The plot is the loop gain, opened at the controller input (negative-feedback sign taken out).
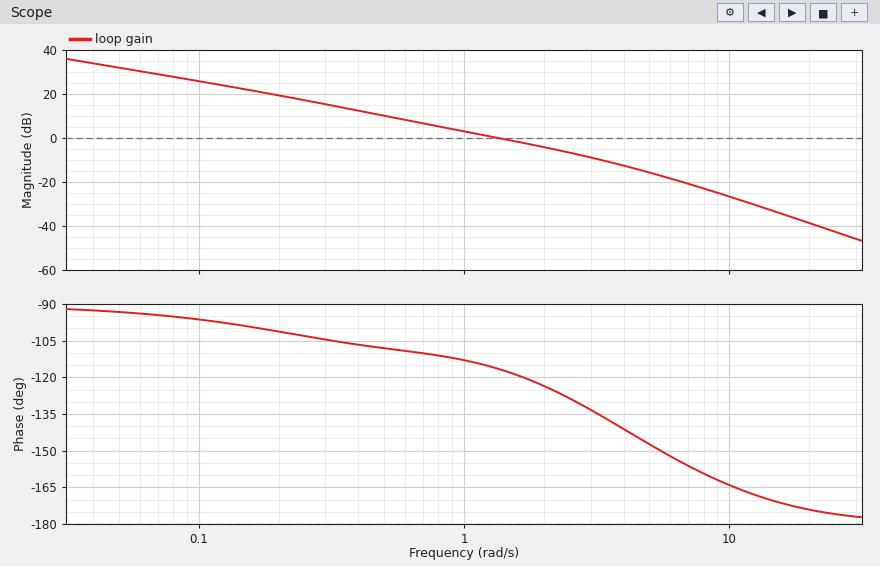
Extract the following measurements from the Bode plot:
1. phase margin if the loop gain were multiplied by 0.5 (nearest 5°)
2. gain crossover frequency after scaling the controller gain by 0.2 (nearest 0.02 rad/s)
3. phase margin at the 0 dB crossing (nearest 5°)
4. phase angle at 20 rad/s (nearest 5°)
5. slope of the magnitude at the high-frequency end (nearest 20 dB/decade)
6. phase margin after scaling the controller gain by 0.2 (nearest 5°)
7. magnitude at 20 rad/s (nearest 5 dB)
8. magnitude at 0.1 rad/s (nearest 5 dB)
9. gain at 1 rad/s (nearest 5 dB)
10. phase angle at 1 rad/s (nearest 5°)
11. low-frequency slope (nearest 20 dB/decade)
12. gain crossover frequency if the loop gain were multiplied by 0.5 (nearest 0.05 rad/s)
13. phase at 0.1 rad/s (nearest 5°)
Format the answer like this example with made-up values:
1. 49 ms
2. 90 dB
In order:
1. 70°
2. 0.34 rad/s
3. 65°
4. -175°
5. -40 dB/decade
6. 75°
7. -40 dB
8. 25 dB
9. 5 dB
10. -115°
11. -20 dB/decade
12. 0.75 rad/s
13. -95°
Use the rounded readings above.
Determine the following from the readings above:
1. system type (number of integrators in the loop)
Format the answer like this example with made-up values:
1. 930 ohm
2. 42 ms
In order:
1. 1
